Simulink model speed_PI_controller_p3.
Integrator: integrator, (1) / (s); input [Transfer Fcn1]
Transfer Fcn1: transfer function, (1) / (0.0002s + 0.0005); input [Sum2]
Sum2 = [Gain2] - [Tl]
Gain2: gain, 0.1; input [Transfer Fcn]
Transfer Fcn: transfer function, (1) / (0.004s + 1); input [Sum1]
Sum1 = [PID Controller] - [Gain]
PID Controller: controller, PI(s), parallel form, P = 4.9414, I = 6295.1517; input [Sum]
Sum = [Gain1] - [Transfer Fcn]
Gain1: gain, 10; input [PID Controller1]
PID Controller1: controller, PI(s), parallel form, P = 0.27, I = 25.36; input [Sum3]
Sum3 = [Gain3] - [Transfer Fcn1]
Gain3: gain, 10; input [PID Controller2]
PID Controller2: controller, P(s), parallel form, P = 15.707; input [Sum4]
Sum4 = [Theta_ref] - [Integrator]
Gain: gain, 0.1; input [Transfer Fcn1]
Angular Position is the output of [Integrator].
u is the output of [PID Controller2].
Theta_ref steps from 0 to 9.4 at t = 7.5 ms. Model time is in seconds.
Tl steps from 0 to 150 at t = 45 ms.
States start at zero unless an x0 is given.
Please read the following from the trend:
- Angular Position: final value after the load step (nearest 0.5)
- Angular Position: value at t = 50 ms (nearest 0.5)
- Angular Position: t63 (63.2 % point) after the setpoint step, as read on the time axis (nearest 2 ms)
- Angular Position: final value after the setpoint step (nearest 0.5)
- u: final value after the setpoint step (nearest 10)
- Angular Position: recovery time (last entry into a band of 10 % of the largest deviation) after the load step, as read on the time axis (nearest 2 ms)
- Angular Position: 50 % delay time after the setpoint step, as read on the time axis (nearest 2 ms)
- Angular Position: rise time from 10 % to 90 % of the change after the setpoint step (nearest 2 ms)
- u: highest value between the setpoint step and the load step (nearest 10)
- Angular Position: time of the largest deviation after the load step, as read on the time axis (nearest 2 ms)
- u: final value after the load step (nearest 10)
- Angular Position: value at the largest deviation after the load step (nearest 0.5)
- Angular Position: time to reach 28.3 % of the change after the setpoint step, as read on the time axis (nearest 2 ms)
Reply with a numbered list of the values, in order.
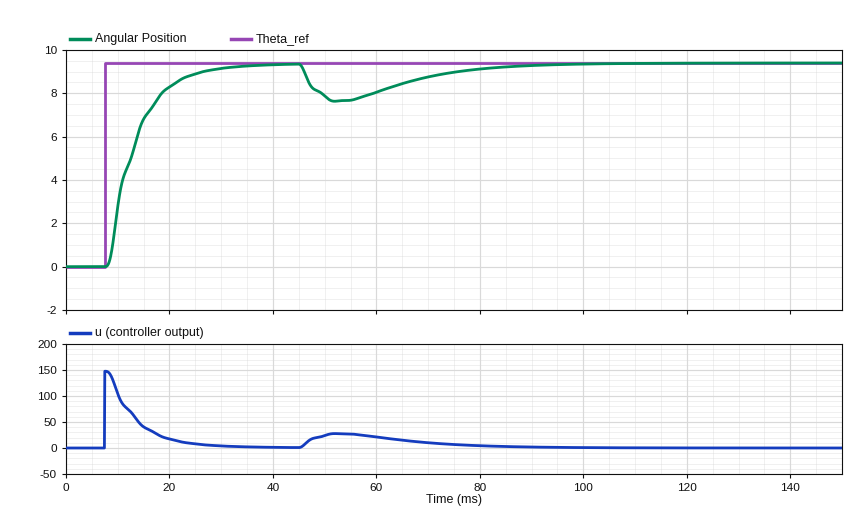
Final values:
1. 9.5
2. 8.0
3. 14 ms
4. 9.5
5. 0
6. 86 ms
7. 12 ms
8. 12 ms
9. 150
10. 52 ms
11. 0
12. 7.5
13. 10 ms
